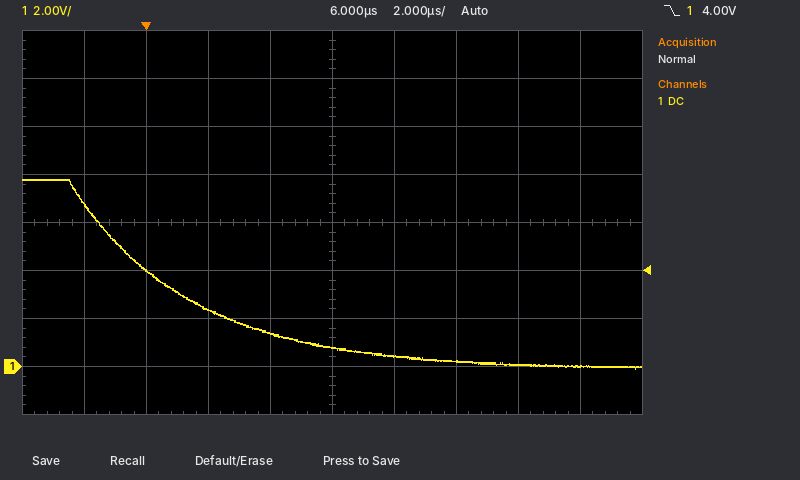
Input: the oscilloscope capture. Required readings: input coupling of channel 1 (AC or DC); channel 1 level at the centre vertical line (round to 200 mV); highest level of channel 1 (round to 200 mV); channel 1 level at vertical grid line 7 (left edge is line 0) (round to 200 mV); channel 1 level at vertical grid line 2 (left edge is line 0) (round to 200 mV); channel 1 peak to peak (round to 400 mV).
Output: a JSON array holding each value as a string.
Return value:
["DC", "800 mV", "7.8 V", "200 mV", "4.0 V", "8.0 V"]
